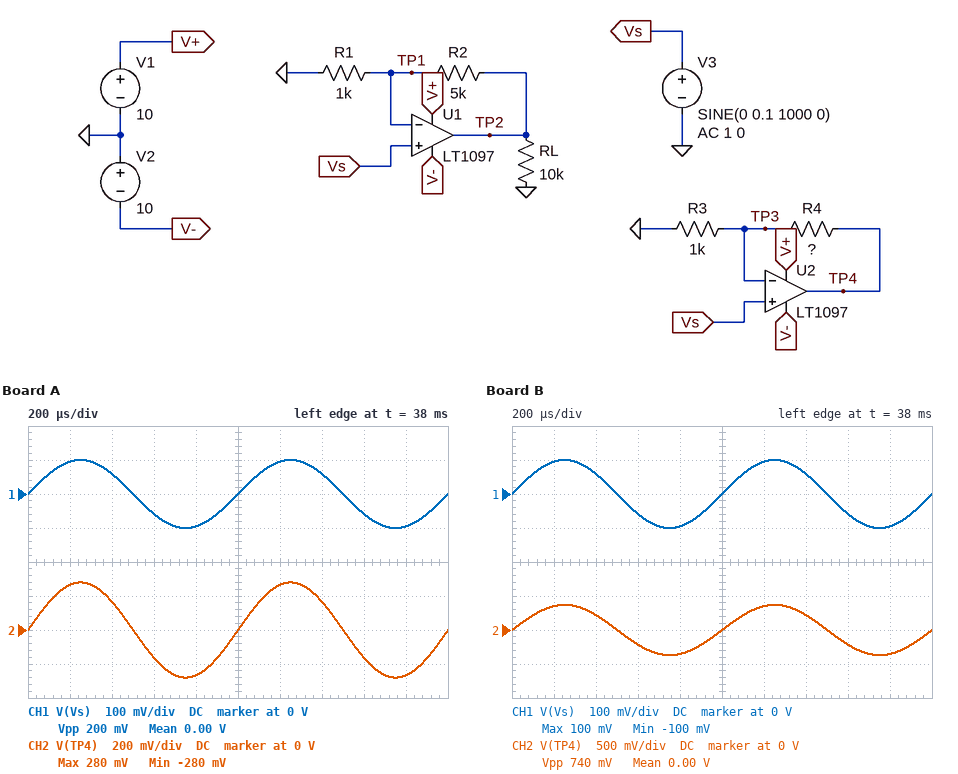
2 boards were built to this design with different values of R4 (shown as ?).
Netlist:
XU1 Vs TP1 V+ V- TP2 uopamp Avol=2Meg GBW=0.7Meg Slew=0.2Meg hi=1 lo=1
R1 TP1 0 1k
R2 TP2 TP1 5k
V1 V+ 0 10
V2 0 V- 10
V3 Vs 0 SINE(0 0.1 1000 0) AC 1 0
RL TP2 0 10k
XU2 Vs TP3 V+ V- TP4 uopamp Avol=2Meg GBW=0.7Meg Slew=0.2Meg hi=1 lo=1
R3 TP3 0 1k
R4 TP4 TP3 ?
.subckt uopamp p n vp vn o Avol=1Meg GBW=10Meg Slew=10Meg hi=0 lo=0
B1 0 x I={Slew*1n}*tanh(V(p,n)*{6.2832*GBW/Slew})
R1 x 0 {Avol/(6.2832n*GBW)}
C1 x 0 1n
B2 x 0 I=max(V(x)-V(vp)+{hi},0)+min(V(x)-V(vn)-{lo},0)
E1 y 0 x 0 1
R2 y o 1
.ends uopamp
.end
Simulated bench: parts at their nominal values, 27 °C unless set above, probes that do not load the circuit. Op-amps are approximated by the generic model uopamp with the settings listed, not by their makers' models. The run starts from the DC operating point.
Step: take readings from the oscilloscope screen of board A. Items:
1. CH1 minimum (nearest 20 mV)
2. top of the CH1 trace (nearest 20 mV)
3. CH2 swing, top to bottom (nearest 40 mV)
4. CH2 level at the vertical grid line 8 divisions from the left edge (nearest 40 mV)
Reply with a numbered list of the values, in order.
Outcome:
1. -100 mV
2. 100 mV
3. 560 mV
4. -160 mV
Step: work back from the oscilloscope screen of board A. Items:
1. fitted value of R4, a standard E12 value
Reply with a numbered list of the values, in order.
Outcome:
1. 1.8 kΩ
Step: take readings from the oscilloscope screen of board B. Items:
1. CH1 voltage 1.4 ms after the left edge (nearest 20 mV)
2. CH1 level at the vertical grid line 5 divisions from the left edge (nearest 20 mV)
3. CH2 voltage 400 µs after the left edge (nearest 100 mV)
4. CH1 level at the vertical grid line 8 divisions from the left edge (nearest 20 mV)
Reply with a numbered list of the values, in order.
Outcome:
1. 60 mV
2. 0 V
3. 200 mV
4. -60 mV
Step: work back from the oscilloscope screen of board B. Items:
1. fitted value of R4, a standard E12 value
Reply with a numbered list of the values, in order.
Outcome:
1. 2.7 kΩ
